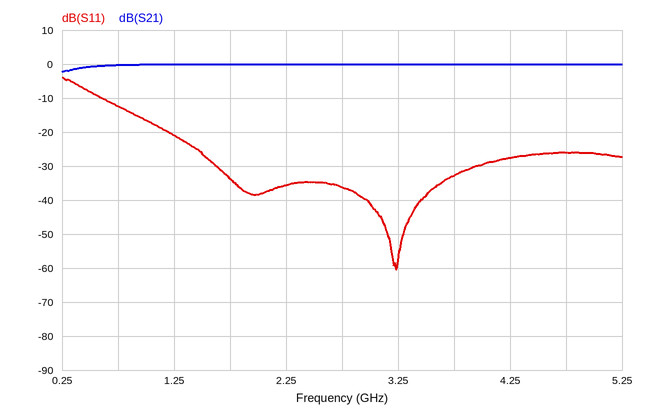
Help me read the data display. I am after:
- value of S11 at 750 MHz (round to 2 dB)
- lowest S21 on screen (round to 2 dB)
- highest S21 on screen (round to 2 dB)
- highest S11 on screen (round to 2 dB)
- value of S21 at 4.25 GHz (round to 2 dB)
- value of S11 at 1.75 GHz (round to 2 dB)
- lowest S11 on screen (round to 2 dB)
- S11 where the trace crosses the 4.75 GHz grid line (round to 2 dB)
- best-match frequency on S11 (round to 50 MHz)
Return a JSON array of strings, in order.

["-12 dB", "-2 dB", "0 dB", "-4 dB", "0 dB", "-34 dB", "-60 dB", "-26 dB", "3.25 GHz"]
